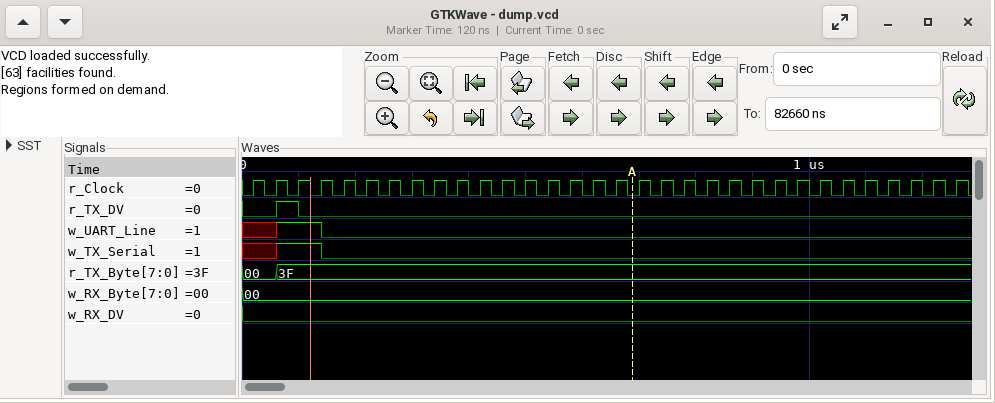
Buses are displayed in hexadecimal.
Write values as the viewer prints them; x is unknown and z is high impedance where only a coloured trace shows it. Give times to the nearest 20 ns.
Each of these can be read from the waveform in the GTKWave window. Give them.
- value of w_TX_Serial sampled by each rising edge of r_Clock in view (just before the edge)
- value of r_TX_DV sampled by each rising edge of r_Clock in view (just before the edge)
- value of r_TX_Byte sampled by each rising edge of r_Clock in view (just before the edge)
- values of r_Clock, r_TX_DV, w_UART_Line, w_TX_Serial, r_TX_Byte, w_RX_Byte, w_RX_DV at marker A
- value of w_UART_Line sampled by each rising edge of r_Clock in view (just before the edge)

x x 1 1 0 0 0 0 0 0 0 0 0 0 0 0 0 0 0 0 0 0 0 0 0 0 0 0 0 0 0 0
0 0 1 0 0 0 0 0 0 0 0 0 0 0 0 0 0 0 0 0 0 0 0 0 0 0 0 0 0 0 0 0
00, 00, 3F, 3F, 3F, 3F, 3F, 3F, 3F, 3F, 3F, 3F, 3F, 3F, 3F, 3F, 3F, 3F, 3F, 3F, 3F, 3F, 3F, 3F, 3F, 3F, 3F, 3F, 3F, 3F, 3F, 3F
r_Clock=0, r_TX_DV=0, w_UART_Line=0, w_TX_Serial=0, r_TX_Byte=3F, w_RX_Byte=00, w_RX_DV=0
x x 1 1 0 0 0 0 0 0 0 0 0 0 0 0 0 0 0 0 0 0 0 0 0 0 0 0 0 0 0 0
